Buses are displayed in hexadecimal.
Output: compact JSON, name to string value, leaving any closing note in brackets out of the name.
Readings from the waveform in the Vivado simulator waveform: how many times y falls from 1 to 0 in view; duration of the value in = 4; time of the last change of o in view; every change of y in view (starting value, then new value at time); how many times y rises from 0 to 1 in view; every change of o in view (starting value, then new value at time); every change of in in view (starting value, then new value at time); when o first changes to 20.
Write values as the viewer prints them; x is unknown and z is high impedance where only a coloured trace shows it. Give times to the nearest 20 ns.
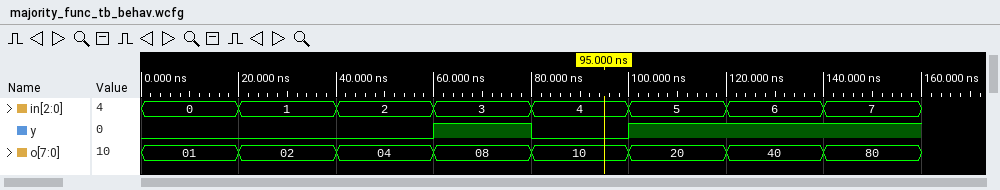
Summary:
{"how many times y falls from 1 to 0 in view": "1", "duration of the value in = 4": "20 ns", "time of the last change of o in view": "140 ns", "every change of y in view": "0, 1 at 60 ns, 0 at 80 ns, 1 at 100 ns", "how many times y rises from 0 to 1 in view": "2", "every change of o in view": "01, 02 at 20 ns, 04 at 40 ns, 08 at 60 ns, 10 at 80 ns, 20 at 100 ns, 40 at 120 ns, 80 at 140 ns", "every change of in in view": "0, 1 at 20 ns, 2 at 40 ns, 3 at 60 ns, 4 at 80 ns, 5 at 100 ns, 6 at 120 ns, 7 at 140 ns", "when o first changes to 20": "100 ns"}
